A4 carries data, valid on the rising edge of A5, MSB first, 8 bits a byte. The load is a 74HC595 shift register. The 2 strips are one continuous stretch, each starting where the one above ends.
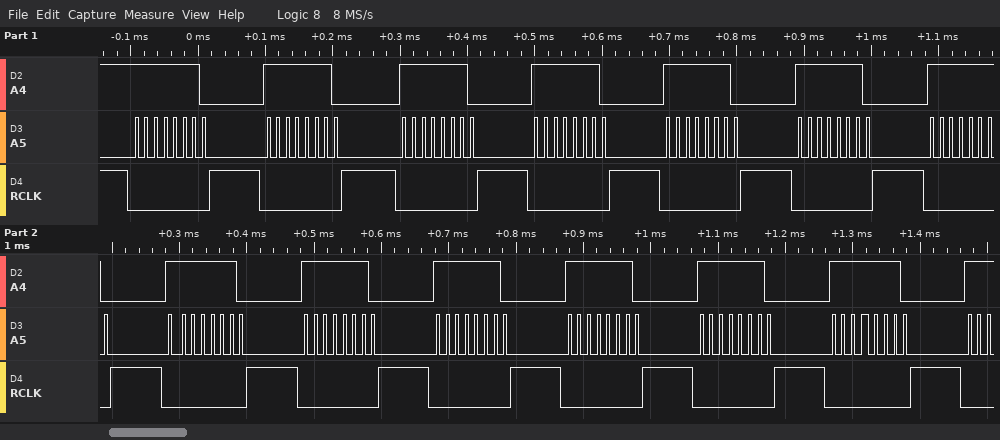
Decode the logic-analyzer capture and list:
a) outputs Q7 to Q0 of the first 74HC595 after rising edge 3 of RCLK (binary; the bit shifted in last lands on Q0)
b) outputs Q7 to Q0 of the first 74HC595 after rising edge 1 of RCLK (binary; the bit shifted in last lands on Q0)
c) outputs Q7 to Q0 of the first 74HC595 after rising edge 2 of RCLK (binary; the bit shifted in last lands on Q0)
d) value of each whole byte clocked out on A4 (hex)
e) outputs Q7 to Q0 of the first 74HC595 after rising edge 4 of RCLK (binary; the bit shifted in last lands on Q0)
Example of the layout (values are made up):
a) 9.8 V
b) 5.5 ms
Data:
a) 11111110
b) 11111110
c) 11111110
d) FE FE FE FE FE FE FE FE FE FE FE FE FE
e) 11111110
